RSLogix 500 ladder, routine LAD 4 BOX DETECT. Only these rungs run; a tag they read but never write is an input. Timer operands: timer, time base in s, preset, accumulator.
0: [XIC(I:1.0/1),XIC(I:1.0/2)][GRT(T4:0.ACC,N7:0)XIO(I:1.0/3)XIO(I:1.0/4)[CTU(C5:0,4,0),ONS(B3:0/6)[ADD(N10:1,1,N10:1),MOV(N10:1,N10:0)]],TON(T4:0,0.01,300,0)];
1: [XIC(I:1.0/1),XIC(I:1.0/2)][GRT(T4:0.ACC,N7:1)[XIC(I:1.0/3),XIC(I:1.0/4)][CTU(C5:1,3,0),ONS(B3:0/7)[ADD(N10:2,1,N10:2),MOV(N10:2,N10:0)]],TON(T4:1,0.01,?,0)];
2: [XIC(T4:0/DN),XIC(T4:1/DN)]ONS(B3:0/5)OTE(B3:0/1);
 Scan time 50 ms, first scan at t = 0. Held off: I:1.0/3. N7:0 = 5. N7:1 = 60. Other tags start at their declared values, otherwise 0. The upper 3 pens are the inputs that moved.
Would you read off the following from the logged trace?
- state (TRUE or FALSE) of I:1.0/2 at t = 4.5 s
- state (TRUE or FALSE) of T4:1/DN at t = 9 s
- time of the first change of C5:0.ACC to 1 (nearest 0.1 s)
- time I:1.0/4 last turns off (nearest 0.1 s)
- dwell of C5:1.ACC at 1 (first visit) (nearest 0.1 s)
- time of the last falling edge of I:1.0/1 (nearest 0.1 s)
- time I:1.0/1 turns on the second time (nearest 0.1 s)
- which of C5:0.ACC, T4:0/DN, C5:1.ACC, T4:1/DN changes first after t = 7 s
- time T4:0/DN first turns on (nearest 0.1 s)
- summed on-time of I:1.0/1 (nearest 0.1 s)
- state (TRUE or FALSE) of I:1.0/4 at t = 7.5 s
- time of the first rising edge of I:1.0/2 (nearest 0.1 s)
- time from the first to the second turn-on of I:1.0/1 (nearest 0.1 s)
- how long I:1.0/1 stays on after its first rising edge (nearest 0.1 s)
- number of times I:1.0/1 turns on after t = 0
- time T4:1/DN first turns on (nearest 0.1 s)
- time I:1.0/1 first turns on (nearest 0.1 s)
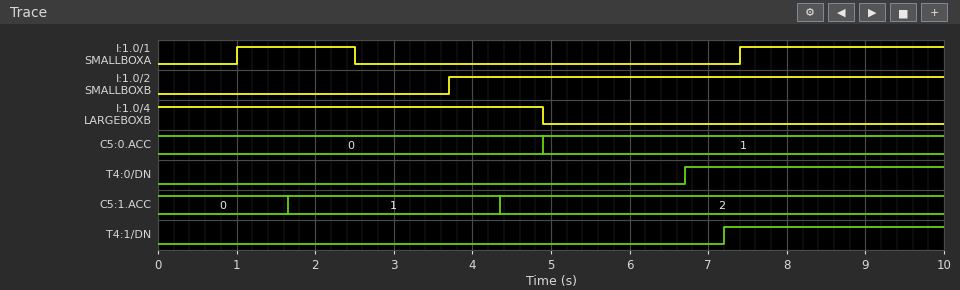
TRUE
TRUE
4.9 s
4.9 s
2.7 s
2.5 s
7.4 s
T4:1/DN
6.7 s
4.1 s
FALSE
3.7 s
6.4 s
1.5 s
2
7.2 s
1.0 s
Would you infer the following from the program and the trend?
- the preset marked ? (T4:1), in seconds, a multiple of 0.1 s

3.5 s
